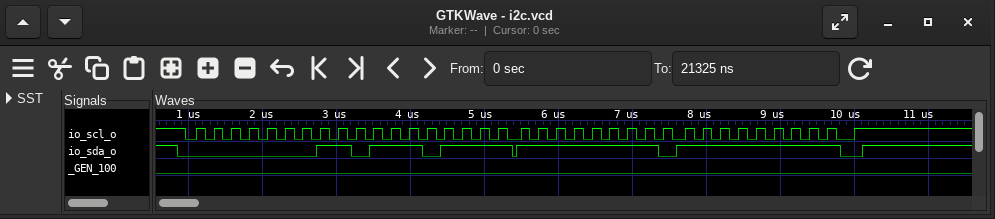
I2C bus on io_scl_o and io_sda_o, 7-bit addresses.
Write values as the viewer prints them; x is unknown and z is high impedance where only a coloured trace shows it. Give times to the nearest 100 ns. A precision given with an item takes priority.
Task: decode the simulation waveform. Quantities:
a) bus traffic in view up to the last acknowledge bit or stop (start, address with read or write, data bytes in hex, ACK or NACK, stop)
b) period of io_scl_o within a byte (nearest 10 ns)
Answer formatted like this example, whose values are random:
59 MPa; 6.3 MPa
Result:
start, address 00 read NACK, 77 NACK, FF ACK, FF NACK, stop; 240 ns
